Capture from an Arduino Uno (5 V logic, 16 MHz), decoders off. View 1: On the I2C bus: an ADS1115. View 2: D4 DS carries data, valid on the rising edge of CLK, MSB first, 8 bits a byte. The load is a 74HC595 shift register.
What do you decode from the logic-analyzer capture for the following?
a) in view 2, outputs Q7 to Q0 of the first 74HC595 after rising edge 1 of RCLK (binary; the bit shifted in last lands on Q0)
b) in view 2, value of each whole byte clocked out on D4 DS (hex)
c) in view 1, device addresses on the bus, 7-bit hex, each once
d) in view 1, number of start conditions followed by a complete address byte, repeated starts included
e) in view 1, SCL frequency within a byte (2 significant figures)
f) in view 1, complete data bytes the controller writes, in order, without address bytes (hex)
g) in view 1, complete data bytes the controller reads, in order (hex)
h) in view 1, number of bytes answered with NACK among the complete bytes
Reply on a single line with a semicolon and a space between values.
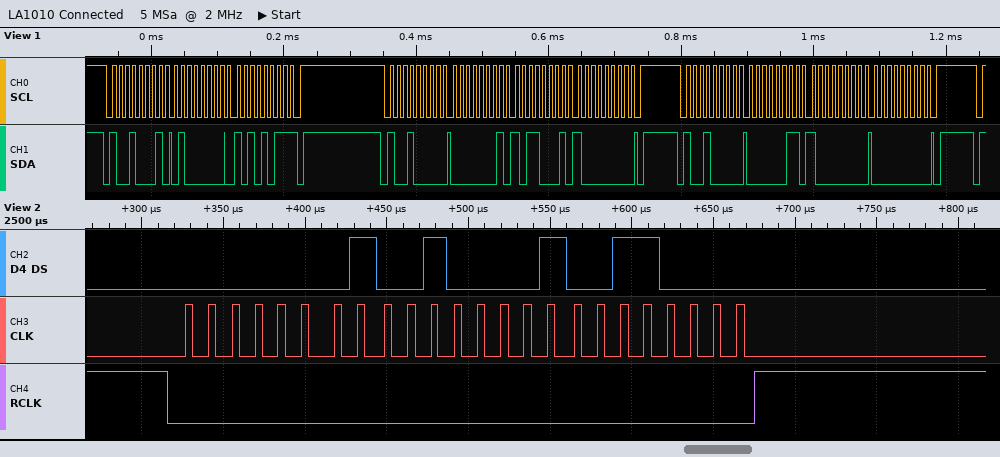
00110000; 0x01 0x21 0x30; 0x48; 3; 100 kHz; 01 B1 80 03 80 00; 40 AB; 1
